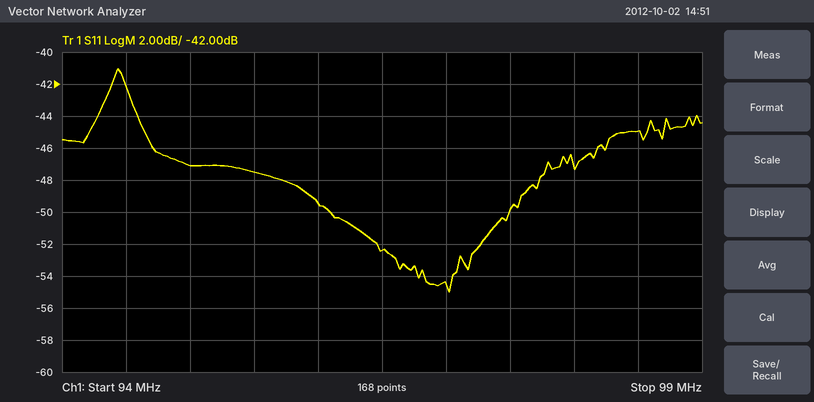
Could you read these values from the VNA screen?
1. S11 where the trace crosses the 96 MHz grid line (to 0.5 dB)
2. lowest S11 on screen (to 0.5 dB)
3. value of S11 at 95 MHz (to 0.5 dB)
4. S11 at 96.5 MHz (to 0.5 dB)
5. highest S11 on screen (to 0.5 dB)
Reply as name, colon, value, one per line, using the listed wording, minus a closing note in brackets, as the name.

S11 where the trace crosses the 96 MHz grid line: -49.5 dB
lowest S11 on screen: -55.0 dB
value of S11 at 95 MHz: -47.0 dB
S11 at 96.5 MHz: -52.5 dB
highest S11 on screen: -41.0 dB
